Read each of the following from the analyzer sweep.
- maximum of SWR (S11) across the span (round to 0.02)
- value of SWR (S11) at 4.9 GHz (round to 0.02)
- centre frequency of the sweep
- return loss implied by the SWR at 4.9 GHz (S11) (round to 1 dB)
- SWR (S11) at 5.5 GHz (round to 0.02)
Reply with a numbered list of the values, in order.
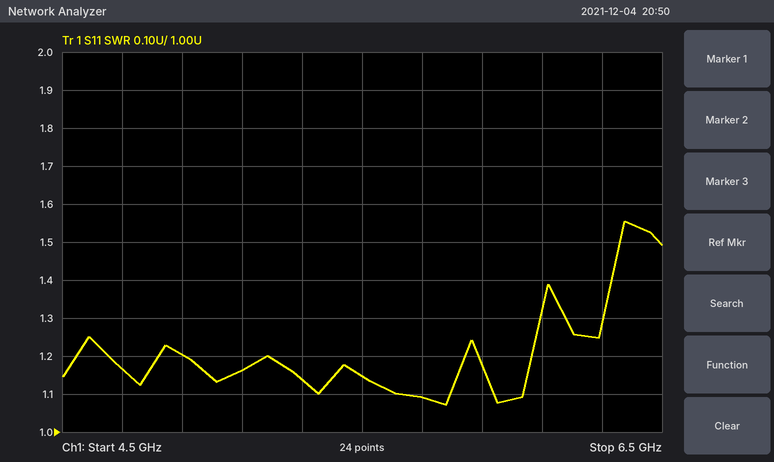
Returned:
1. 1.56
2. 1.20
3. 5.5 GHz
4. 21 dB
5. 1.14
